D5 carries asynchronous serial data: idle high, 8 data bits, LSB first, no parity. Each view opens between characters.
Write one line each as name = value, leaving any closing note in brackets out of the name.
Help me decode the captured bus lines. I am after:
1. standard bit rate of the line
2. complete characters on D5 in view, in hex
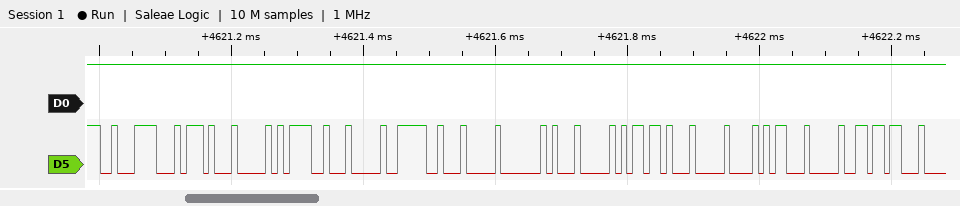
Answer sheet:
standard bit rate of the line = 115200 baud
complete characters on D5 in view, in hex = E2, 74, 04, 3D, 04, 3E, 04, 40, 04, 6D, 04, A8, 04, B6
